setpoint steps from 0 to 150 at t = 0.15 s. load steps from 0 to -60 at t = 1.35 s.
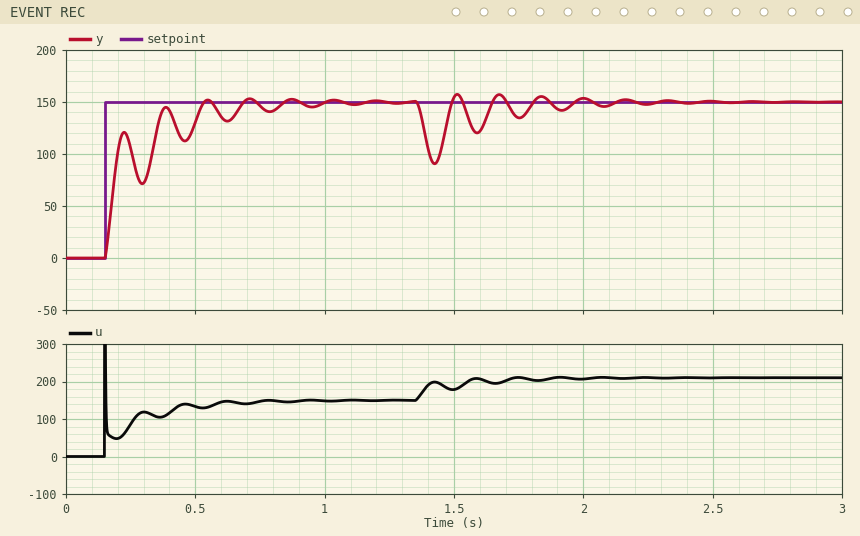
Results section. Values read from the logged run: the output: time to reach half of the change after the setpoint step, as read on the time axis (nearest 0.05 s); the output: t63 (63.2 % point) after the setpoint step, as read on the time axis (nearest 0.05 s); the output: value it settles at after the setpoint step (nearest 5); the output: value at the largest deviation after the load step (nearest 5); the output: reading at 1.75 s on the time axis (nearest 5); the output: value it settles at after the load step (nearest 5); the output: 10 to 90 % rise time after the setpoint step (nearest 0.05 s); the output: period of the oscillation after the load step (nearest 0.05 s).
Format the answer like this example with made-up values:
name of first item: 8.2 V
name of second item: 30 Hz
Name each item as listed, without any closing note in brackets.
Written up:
the output: time to reach half of the change after the setpoint step, as read on the time axis: 0.20 s
the output: t63 (63.2 % point) after the setpoint step, as read on the time axis: 0.20 s
the output: value it settles at after the setpoint step: 150
the output: value at the largest deviation after the load step: 90
the output: reading at 1.75 s on the time axis: 135
the output: value it settles at after the load step: 150
the output: 10 to 90 % rise time after the setpoint step: 0.20 s
the output: period of the oscillation after the load step: 0.15 s
